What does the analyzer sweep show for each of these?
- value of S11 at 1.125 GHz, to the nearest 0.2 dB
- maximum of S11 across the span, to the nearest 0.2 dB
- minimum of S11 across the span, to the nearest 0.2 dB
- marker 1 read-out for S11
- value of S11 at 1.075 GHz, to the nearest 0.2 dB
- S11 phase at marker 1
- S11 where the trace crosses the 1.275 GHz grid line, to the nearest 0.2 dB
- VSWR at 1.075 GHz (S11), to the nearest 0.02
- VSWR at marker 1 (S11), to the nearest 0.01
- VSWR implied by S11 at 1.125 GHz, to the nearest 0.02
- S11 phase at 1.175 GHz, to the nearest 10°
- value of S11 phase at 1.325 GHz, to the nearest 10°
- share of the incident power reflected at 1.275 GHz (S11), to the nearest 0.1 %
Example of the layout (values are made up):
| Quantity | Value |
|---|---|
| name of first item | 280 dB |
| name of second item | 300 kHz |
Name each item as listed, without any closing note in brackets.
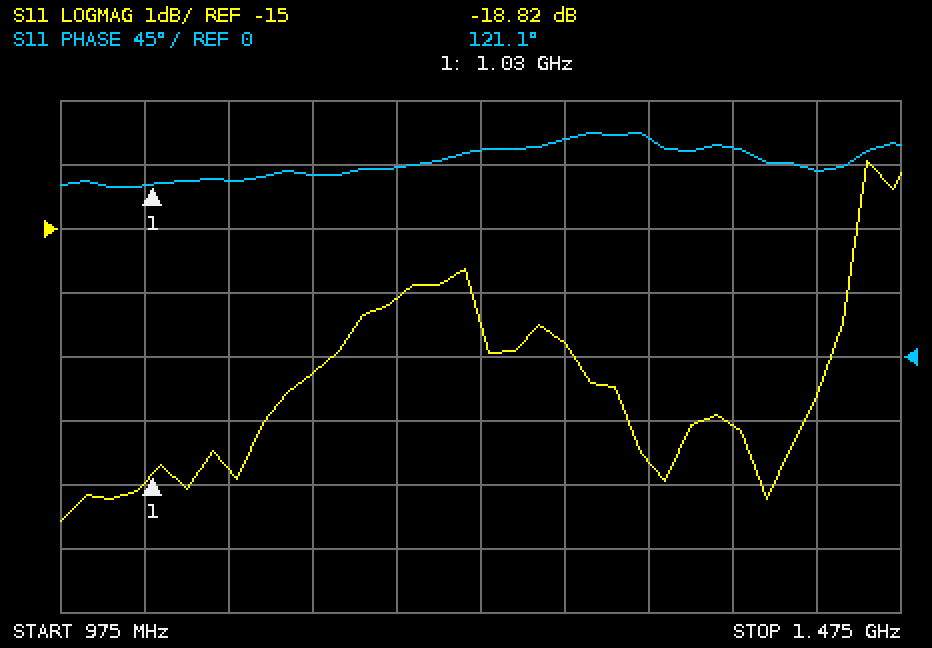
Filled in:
| Quantity | Value |
|---|---|
| value of S11 at 1.125 GHz, to the nearest 0.2 dB | -17.2 dB |
| maximum of S11 across the span, to the nearest 0.2 dB | -14.0 dB |
| minimum of S11 across the span, to the nearest 0.2 dB | -19.6 dB |
| marker 1 read-out for S11 | -18.82 dB |
| value of S11 at 1.075 GHz, to the nearest 0.2 dB | -18.8 dB |
| S11 phase at marker 1 | 121.1° |
| S11 where the trace crosses the 1.275 GHz grid line, to the nearest 0.2 dB | -16.8 dB |
| VSWR at 1.075 GHz (S11), to the nearest 0.02 | 1.26 |
| VSWR at marker 1 (S11), to the nearest 0.01 | 1.26 |
| VSWR implied by S11 at 1.125 GHz, to the nearest 0.02 | 1.32 |
| S11 phase at 1.175 GHz, to the nearest 10° | 130° |
| value of S11 phase at 1.325 GHz, to the nearest 10° | 150° |
| share of the incident power reflected at 1.275 GHz (S11), to the nearest 0.1 % | 2.1 % |
